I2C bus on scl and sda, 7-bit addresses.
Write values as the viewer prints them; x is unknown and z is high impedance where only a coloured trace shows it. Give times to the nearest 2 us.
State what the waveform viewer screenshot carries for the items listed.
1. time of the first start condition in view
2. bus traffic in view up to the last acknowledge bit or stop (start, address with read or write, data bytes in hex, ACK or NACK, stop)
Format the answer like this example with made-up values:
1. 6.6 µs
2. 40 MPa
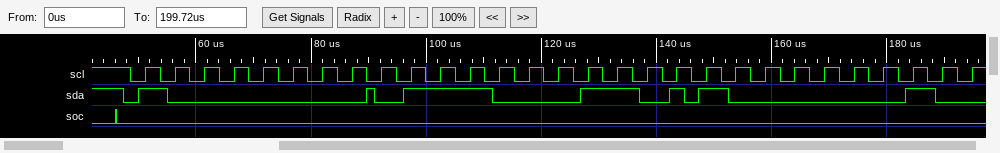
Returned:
1. 48 us
2. start, address 40 write ACK, E3 ACK, repeated start, address 40 read ACK
